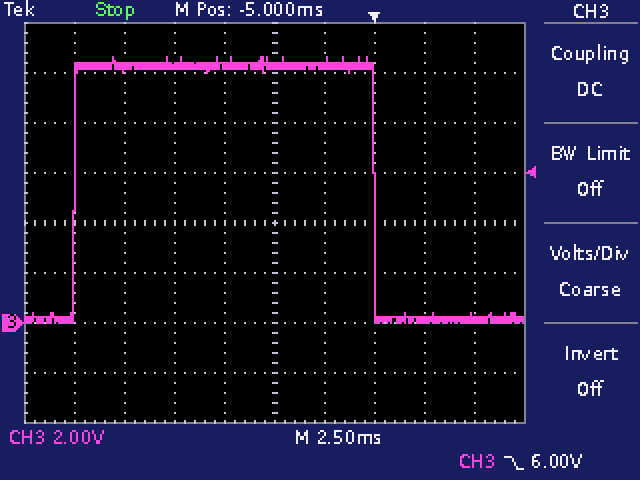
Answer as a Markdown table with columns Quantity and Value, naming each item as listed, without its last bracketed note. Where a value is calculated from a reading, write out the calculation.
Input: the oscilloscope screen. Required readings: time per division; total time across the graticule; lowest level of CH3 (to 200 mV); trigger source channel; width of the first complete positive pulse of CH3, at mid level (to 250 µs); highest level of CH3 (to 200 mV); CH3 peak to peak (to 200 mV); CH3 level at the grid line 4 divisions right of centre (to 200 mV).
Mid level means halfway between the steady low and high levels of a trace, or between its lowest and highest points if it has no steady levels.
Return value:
| Quantity | Value |
|---|---|
| time per division | 2.5 ms |
| total time across the graticule | 25 ms |
| lowest level of CH3 | 0.0 V |
| trigger source channel | CH3 |
| width of the first complete positive pulse of CH3, at mid level | 15.00 ms |
| highest level of CH3 | 10.6 V |
| CH3 peak to peak | 10.6 V − (0.0 V) = 10.6 V |
| CH3 level at the grid line 4 divisions right of centre | 200 mV |
